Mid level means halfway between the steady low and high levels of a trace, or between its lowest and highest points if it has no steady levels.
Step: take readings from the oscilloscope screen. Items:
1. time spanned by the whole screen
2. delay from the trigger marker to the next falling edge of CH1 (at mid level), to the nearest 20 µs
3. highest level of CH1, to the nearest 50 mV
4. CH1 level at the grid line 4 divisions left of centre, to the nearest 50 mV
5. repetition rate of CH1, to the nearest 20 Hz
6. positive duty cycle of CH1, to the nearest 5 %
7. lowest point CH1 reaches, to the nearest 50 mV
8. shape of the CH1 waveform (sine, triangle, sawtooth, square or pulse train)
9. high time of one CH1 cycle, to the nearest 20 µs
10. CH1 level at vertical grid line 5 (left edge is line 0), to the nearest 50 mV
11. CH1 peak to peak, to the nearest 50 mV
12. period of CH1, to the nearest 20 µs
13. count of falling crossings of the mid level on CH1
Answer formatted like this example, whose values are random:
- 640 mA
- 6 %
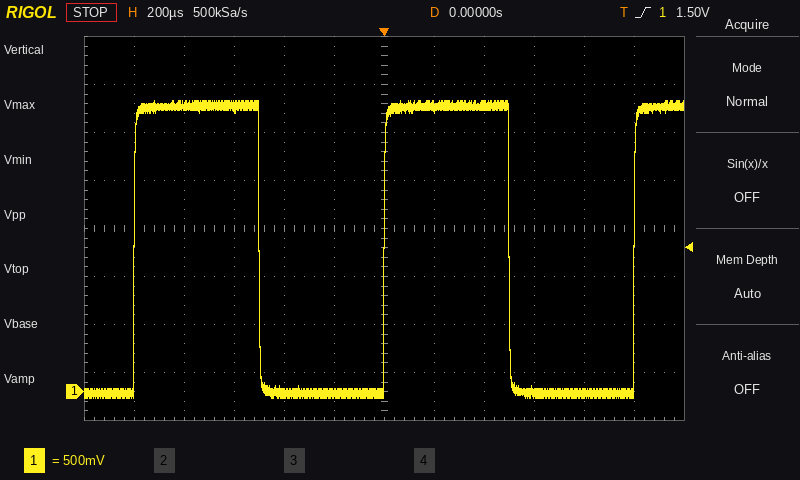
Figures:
- 2.4 ms
- 500 µs
- 3.05 V
- 3.00 V
- 1.00 kHz
- 50 %
- -50 mV
- square
- 500 µs
- 0 mV
- 3.10 V
- 1.00 ms
- 2
